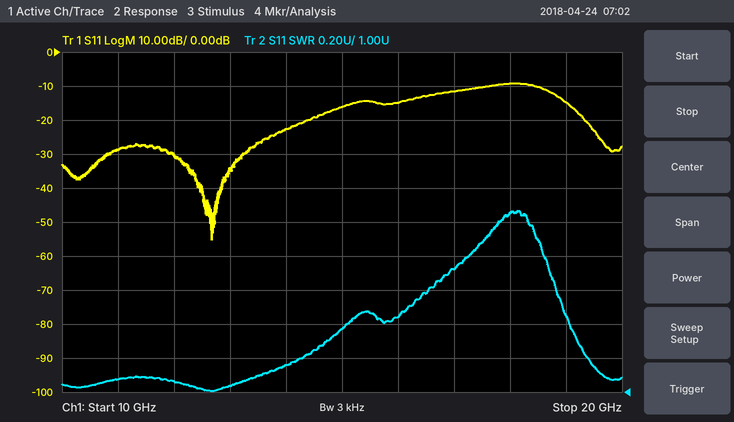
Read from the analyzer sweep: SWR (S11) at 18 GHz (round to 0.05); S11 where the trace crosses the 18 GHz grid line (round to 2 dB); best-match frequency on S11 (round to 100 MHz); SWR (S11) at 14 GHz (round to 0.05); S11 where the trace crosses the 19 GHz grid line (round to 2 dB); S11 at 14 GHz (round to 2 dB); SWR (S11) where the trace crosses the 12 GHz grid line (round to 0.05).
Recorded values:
2.05
-10 dB
12.7 GHz
1.15
-14 dB
-22 dB
1.05
